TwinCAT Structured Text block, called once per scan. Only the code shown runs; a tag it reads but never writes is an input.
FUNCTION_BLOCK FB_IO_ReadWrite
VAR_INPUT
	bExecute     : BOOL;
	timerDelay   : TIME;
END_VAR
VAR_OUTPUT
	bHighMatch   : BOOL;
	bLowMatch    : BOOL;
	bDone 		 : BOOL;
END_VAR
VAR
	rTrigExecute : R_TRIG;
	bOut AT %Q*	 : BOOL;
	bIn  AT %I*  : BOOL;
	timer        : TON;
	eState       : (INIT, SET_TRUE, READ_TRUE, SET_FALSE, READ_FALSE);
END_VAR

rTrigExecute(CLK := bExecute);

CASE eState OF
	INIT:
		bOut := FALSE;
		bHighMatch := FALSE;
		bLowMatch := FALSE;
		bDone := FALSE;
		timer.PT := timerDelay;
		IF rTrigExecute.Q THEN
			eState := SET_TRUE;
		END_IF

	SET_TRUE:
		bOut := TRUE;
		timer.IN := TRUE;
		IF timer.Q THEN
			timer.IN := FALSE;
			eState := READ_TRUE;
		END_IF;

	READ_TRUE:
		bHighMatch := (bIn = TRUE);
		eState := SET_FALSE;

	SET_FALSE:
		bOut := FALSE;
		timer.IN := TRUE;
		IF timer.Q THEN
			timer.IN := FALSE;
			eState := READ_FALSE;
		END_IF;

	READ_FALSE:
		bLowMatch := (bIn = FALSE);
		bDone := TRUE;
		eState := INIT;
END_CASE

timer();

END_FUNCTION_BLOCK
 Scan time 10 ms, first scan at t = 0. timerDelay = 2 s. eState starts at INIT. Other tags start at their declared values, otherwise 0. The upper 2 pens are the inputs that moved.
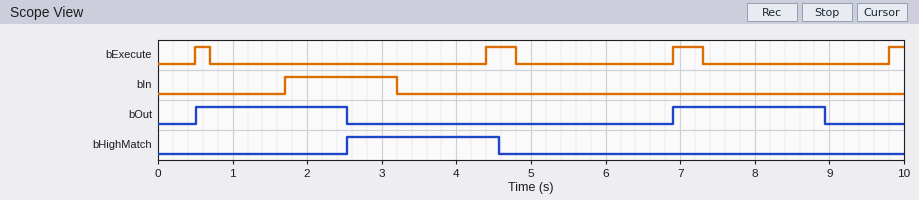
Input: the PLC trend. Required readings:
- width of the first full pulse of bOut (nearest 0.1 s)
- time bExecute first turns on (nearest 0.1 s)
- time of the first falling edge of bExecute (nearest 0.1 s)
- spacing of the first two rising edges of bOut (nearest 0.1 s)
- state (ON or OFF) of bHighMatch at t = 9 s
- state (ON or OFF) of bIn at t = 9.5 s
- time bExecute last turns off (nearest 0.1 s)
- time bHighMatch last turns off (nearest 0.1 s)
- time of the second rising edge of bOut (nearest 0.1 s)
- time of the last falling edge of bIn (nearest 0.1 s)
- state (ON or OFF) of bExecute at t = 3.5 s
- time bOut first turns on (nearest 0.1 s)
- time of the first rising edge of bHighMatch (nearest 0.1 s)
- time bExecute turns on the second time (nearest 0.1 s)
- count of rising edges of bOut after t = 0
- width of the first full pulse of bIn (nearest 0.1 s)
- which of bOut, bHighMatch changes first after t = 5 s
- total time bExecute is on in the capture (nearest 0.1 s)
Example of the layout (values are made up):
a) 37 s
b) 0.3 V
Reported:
a) 2.0 s
b) 0.5 s
c) 0.7 s
d) 6.4 s
e) OFF
f) OFF
g) 7.3 s
h) 4.6 s
i) 6.9 s
j) 3.2 s
k) OFF
l) 0.5 s
m) 2.5 s
n) 4.4 s
o) 2
p) 1.5 s
q) bOut
r) 1.2 s
